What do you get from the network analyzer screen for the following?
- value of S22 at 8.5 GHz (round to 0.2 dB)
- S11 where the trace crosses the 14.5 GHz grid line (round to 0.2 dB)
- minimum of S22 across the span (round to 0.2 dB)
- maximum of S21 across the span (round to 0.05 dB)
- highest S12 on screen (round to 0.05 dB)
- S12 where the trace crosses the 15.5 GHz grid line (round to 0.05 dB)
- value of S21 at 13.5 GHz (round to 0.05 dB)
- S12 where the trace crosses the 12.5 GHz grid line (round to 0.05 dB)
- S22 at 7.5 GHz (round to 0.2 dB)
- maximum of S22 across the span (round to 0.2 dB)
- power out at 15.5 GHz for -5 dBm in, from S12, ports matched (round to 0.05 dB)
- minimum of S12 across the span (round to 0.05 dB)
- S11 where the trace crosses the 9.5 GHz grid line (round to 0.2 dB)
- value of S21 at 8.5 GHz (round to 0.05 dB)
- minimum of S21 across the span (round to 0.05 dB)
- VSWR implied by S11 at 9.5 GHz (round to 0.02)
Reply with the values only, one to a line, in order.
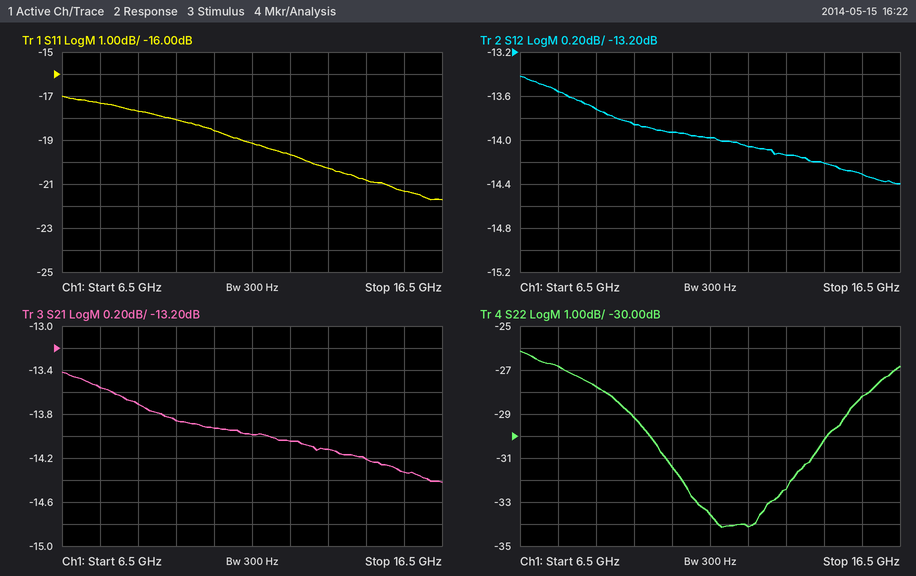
-27.8 dB
-20.8 dB
-34.2 dB
-13.40 dB
-13.40 dB
-14.30 dB
-14.10 dB
-14.05 dB
-26.8 dB
-26.2 dB
-19.30 dBm
-14.40 dB
-18.0 dB
-13.70 dB
-14.40 dB
1.28
